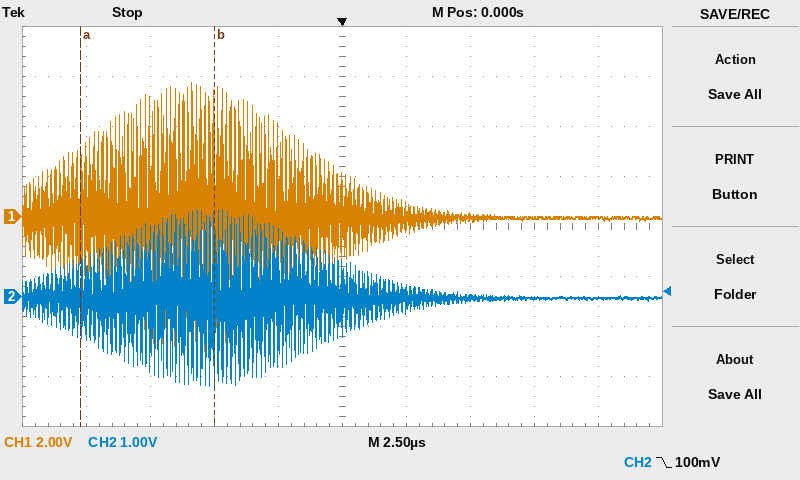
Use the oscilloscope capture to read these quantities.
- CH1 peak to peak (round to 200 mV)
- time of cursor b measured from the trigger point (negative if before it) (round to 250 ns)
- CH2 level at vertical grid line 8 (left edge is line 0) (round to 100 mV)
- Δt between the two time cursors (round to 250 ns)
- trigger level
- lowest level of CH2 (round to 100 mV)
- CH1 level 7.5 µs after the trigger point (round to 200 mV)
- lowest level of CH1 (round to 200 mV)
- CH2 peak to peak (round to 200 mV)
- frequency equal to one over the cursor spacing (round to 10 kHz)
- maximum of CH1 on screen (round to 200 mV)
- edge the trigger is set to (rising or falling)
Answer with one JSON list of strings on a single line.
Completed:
["10.8 V", "-5.00 µs", "0.0 V", "5.25 µs", "100 mV", "-1.8 V", "0.0 V", "-5.4 V", "3.6 V", "190 kHz", "5.4 V", "falling"]
